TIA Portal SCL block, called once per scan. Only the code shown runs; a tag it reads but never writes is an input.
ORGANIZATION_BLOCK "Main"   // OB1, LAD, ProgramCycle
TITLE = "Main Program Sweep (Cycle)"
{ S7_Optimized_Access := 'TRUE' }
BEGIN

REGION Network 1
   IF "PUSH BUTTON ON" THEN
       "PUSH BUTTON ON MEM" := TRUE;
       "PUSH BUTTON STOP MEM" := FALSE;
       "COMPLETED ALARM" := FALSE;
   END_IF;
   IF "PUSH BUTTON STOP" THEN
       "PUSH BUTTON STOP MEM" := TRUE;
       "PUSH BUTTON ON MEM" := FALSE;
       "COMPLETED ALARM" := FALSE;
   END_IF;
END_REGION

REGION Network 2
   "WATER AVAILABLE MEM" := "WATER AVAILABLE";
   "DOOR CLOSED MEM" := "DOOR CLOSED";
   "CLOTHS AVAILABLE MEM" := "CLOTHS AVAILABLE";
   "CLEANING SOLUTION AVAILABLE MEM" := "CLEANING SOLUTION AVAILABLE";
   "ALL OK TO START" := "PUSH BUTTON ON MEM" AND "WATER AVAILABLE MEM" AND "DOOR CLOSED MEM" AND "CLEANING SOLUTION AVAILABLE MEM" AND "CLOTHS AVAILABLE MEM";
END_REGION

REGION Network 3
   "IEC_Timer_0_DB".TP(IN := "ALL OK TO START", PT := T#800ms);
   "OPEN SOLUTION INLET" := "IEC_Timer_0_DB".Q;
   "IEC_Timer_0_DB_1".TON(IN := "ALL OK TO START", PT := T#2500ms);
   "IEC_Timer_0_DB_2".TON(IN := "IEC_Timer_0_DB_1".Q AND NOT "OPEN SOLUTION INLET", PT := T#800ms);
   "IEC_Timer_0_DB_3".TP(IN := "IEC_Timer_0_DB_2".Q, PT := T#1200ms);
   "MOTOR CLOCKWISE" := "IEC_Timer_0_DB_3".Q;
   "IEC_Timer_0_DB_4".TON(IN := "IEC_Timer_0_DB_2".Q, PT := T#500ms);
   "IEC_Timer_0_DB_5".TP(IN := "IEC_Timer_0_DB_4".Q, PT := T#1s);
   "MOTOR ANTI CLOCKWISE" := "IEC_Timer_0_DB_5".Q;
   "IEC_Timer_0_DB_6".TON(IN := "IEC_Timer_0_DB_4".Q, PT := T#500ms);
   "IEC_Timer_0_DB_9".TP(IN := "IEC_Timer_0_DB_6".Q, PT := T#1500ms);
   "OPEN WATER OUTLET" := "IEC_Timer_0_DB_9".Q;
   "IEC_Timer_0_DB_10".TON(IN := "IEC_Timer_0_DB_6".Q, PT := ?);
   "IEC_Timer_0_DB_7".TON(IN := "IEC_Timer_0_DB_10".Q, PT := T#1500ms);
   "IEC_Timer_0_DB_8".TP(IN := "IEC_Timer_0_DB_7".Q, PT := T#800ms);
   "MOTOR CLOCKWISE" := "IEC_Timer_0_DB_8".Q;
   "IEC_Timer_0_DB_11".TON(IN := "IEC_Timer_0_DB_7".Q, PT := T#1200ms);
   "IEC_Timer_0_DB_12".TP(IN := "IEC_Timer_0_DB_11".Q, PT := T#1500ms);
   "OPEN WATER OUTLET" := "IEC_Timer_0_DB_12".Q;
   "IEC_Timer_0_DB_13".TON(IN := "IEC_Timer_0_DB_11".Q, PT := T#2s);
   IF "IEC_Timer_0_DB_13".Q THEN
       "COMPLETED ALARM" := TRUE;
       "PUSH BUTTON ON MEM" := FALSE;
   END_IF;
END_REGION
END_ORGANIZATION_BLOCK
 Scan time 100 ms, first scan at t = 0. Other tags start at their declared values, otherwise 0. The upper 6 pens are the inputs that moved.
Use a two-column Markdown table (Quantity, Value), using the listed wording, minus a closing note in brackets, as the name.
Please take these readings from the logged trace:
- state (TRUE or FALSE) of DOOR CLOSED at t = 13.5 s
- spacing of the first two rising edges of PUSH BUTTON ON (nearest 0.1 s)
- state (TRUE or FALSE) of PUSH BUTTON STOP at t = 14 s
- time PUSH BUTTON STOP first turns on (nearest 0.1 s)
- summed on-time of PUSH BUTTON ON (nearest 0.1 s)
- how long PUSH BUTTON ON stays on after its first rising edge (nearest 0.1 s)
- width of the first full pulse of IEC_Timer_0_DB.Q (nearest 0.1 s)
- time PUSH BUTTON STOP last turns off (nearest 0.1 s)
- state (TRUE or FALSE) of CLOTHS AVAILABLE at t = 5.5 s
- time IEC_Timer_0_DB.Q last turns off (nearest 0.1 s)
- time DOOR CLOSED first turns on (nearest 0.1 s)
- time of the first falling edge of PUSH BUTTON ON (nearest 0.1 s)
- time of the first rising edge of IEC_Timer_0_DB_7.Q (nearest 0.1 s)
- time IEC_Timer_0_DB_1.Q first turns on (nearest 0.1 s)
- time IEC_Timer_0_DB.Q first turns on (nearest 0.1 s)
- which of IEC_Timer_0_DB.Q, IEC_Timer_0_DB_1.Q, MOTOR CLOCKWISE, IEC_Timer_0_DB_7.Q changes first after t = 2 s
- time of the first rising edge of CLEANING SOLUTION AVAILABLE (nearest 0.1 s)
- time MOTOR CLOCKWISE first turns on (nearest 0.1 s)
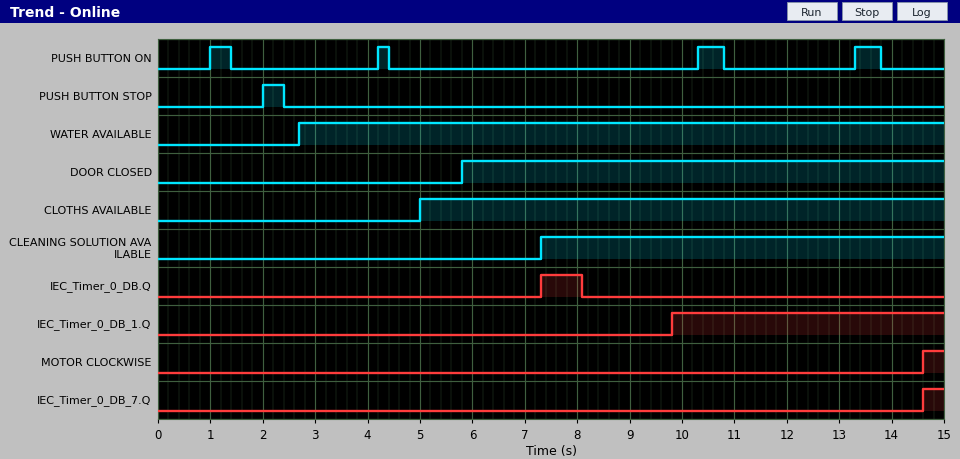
| Quantity | Value |
|---|---|
| state (TRUE or FALSE) of DOOR CLOSED at t = 13.5 s | TRUE |
| spacing of the first two rising edges of PUSH BUTTON ON | 3.2 s |
| state (TRUE or FALSE) of PUSH BUTTON STOP at t = 14 s | FALSE |
| time PUSH BUTTON STOP first turns on | 2.0 s |
| summed on-time of PUSH BUTTON ON | 1.6 s |
| how long PUSH BUTTON ON stays on after its first rising edge | 0.4 s |
| width of the first full pulse of IEC_Timer_0_DB.Q | 0.8 s |
| time PUSH BUTTON STOP last turns off | 2.4 s |
| state (TRUE or FALSE) of CLOTHS AVAILABLE at t = 5.5 s | TRUE |
| time IEC_Timer_0_DB.Q last turns off | 8.1 s |
| time DOOR CLOSED first turns on | 5.8 s |
| time of the first falling edge of PUSH BUTTON ON | 1.4 s |
| time of the first rising edge of IEC_Timer_0_DB_7.Q | 14.6 s |
| time IEC_Timer_0_DB_1.Q first turns on | 9.8 s |
| time IEC_Timer_0_DB.Q first turns on | 7.3 s |
| which of IEC_Timer_0_DB.Q, IEC_Timer_0_DB_1.Q, MOTOR CLOCKWISE, IEC_Timer_0_DB_7.Q changes first after t = 2 s | IEC_Timer_0_DB.Q |
| time of the first rising edge of CLEANING SOLUTION AVAILABLE | 7.3 s |
| time MOTOR CLOCKWISE first turns on | 14.6 s |
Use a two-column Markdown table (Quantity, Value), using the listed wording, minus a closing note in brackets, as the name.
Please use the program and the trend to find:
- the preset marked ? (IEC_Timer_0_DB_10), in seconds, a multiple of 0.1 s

| Quantity | Value |
|---|---|
| the preset marked ? (IEC_Timer_0_DB_10), in seconds, a multiple of 0.1 s | 1.5 s |
